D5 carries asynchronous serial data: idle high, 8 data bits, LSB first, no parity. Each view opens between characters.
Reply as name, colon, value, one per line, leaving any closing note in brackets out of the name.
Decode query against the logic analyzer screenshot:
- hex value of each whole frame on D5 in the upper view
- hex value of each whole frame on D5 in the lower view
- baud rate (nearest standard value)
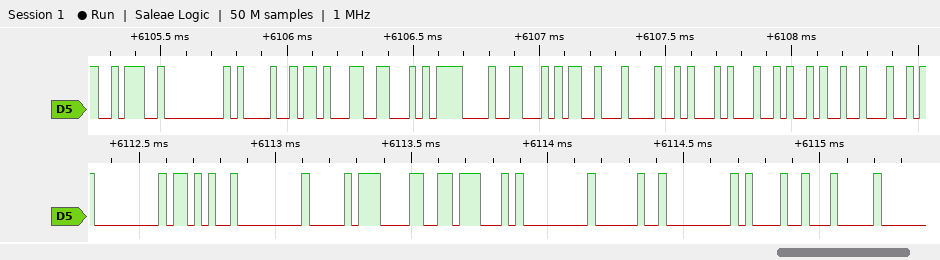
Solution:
hex value of each whole frame on D5 in the upper view: 3A, 00, 21, 8B, 46, 0F, 46, 13, 48, 14, 4A, 12
hex value of each whole frame on D5 in the lower view: 00, 2B, 00, D0, 98, 47, 00, 20, 00, 21, 04
baud rate: 38400 baud
